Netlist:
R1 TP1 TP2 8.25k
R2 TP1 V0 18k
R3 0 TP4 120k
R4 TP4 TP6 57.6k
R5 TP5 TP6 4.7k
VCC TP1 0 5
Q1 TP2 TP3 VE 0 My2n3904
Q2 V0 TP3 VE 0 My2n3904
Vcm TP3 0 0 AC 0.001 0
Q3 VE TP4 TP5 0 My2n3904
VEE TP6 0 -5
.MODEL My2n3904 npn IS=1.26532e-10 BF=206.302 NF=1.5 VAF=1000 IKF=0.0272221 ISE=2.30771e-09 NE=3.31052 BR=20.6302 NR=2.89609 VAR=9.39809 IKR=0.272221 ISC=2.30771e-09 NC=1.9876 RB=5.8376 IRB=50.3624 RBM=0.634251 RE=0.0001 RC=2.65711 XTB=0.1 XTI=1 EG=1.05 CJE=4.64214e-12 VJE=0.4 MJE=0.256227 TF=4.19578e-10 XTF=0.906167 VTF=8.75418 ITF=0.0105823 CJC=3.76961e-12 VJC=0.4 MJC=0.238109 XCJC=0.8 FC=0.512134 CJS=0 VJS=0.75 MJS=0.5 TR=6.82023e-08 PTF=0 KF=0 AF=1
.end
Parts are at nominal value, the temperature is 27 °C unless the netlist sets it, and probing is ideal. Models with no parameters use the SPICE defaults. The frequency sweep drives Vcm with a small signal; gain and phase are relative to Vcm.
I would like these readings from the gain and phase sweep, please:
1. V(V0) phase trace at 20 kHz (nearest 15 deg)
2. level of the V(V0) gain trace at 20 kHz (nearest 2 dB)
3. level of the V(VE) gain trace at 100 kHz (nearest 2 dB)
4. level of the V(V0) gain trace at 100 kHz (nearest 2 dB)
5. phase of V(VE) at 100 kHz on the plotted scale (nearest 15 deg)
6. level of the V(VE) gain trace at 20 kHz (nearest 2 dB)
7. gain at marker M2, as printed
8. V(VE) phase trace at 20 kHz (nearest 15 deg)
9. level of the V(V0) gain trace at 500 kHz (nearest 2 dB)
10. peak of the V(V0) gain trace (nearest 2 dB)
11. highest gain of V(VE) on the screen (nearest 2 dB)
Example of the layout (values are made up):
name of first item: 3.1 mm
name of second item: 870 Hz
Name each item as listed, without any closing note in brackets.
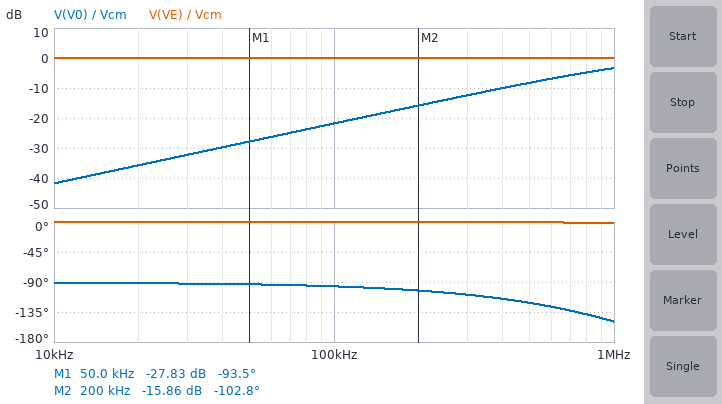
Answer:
V(V0) phase trace at 20 kHz: -90 deg
level of the V(V0) gain trace at 20 kHz: -36 dB
level of the V(VE) gain trace at 100 kHz: 0 dB
level of the V(V0) gain trace at 100 kHz: -22 dB
phase of V(VE) at 100 kHz on the plotted scale: 0 deg
level of the V(VE) gain trace at 20 kHz: 0 dB
gain at marker M2, as printed: -15.86 dB
V(VE) phase trace at 20 kHz: 0 deg
level of the V(V0) gain trace at 500 kHz: -8 dB
peak of the V(V0) gain trace: -4 dB
highest gain of V(VE) on the screen: 0 dB
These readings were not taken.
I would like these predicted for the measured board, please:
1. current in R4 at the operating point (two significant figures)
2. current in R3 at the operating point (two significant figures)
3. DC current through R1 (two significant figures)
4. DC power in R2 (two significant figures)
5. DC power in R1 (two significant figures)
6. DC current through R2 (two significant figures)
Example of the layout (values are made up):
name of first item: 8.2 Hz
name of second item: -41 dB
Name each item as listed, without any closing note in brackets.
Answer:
current in R4 at the operating point: 26 µA
current in R3 at the operating point: 29 µA
DC current through R1: 100 µA
DC power in R2: 180 µW
DC power in R1: 82 µW
DC current through R2: 100 µA
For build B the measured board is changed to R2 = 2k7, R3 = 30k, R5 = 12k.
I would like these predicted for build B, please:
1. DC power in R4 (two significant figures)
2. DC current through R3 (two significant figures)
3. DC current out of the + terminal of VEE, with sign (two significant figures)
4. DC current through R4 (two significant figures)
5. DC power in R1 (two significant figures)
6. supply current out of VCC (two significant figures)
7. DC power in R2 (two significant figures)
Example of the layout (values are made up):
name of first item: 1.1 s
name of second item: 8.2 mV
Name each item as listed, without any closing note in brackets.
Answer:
DC power in R4: 180 µW
DC current through R3: 59 µA
DC current out of the + terminal of VEE, with sign: -280 µA
DC current through R4: 56 µA
DC power in R1: 97 µW
supply current out of VCC: 220 µA
DC power in R2: 32 µW
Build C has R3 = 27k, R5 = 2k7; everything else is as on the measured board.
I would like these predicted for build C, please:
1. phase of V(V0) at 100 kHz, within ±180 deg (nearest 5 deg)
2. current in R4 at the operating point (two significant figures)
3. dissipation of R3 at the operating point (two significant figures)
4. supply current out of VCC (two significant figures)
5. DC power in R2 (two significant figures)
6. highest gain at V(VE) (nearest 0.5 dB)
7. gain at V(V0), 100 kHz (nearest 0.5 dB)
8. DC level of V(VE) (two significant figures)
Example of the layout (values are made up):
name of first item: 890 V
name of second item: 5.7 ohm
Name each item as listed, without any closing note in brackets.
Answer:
phase of V(V0) at 100 kHz, within ±180 deg: 0 deg
current in R4 at the operating point: 56 µA
dissipation of R3 at the operating point: 110 µW
supply current out of VCC: 790 µA
DC power in R2: 1.7 mW
highest gain at V(VE): 0 dB
gain at V(V0), 100 kHz: 0 dB
DC level of V(VE): -590 mV
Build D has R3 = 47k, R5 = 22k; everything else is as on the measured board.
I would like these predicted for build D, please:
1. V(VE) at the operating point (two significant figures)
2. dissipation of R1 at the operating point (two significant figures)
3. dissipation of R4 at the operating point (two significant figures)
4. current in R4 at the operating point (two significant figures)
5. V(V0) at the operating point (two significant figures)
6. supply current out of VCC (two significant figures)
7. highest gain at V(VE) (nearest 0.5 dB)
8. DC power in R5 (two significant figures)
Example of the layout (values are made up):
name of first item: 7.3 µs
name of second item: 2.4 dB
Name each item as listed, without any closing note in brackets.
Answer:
V(VE) at the operating point: -500 mV
dissipation of R1 at the operating point: 19 µW
dissipation of R4 at the operating point: 130 µW
current in R4 at the operating point: 47 µA
V(V0) at the operating point: 4.1 V
supply current out of VCC: 96 µA
highest gain at V(VE): 0 dB
DC power in R5: 220 µW
